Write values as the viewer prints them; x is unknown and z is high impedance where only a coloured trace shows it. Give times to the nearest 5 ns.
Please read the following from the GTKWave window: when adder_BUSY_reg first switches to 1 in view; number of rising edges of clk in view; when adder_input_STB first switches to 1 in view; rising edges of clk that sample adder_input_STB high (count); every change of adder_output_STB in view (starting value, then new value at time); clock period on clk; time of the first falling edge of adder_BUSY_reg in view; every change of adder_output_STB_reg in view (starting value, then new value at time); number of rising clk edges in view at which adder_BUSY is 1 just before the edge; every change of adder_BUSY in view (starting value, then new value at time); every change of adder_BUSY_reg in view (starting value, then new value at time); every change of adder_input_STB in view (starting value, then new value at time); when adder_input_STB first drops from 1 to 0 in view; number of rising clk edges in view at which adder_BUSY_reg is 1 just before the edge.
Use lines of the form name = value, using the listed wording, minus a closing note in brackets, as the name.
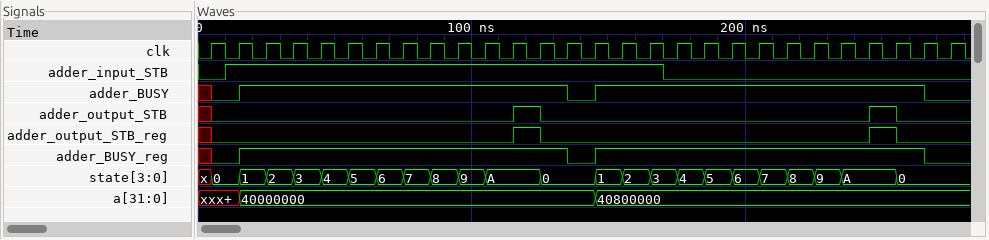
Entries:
when adder_BUSY_reg first switches to 1 in view = 15 ns
number of rising edges of clk in view = 28
when adder_input_STB first switches to 1 in view = 10 ns
rising edges of clk that sample adder_input_STB high = 16
every change of adder_output_STB in view = x, 0 at 5 ns, 1 at 115 ns, 0 at 125 ns, 1 at 245 ns, 0 at 255 ns
clock period on clk = 10 ns
time of the first falling edge of adder_BUSY_reg in view = 135 ns
every change of adder_output_STB_reg in view = x, 0 at 5 ns, 1 at 115 ns, 0 at 125 ns, 1 at 245 ns, 0 at 255 ns
number of rising clk edges in view at which adder_BUSY is 1 just before the edge = 24
every change of adder_BUSY in view = x, 0 at 5 ns, 1 at 15 ns, 0 at 135 ns, 1 at 145 ns, 0 at 265 ns
every change of adder_BUSY_reg in view = x, 0 at 5 ns, 1 at 15 ns, 0 at 135 ns, 1 at 145 ns, 0 at 265 ns
every change of adder_input_STB in view = 0, 1 at 10 ns, 0 at 170 ns
when adder_input_STB first drops from 1 to 0 in view = 170 ns
number of rising clk edges in view at which adder_BUSY_reg is 1 just before the edge = 24
